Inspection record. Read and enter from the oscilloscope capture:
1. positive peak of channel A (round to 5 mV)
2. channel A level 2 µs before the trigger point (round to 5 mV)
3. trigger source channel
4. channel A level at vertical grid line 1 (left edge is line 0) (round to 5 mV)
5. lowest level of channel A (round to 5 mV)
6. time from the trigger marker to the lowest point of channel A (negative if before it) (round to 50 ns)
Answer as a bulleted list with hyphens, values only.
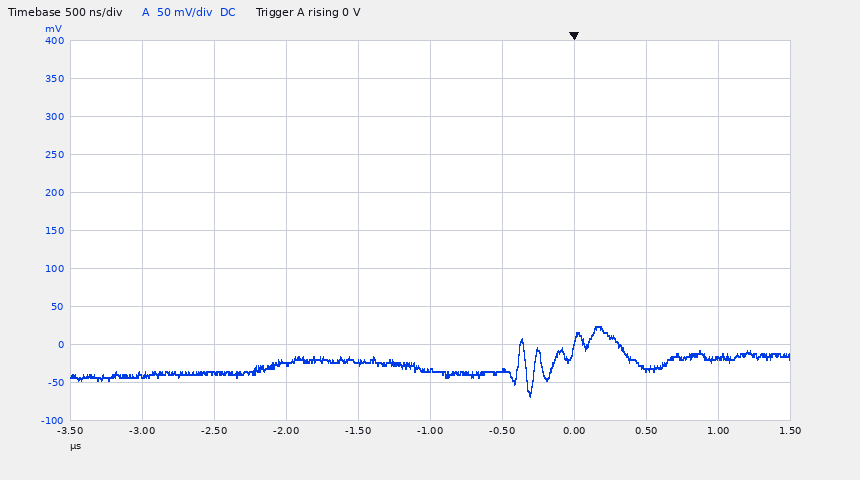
- 25 mV
- -25 mV
- channel A
- -40 mV
- -70 mV
- -300 ns
